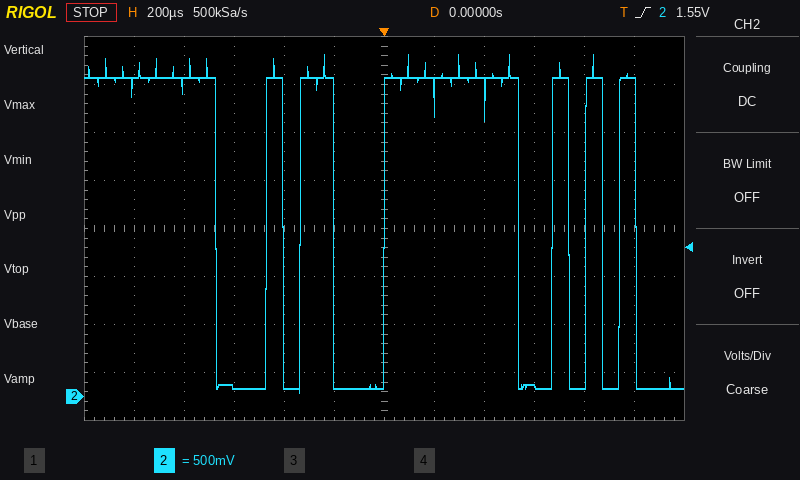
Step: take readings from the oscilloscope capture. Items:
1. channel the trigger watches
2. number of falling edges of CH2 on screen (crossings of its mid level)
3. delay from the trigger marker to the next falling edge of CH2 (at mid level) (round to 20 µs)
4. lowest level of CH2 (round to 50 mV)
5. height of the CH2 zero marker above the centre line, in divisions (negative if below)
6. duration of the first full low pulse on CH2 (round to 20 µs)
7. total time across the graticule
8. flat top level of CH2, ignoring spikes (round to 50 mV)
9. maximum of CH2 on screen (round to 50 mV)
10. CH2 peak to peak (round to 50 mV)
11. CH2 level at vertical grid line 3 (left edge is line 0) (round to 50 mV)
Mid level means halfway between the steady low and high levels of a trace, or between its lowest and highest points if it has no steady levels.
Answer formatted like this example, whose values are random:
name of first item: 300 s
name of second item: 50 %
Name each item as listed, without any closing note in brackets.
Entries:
channel the trigger watches: CH2
number of falling edges of CH2 on screen: 7
delay from the trigger marker to the next falling edge of CH2 (at mid level): 540 µs
lowest level of CH2: 50 mV
height of the CH2 zero marker above the centre line, in divisions: -3.5 div
duration of the first full low pulse on CH2: 200 µs
total time across the graticule: 2.4 ms
flat top level of CH2, ignoring spikes: 3.30 V
maximum of CH2 on screen: 3.55 V
CH2 peak to peak: 3.50 V
CH2 level at vertical grid line 3 (left edge is line 0): 100 mV
